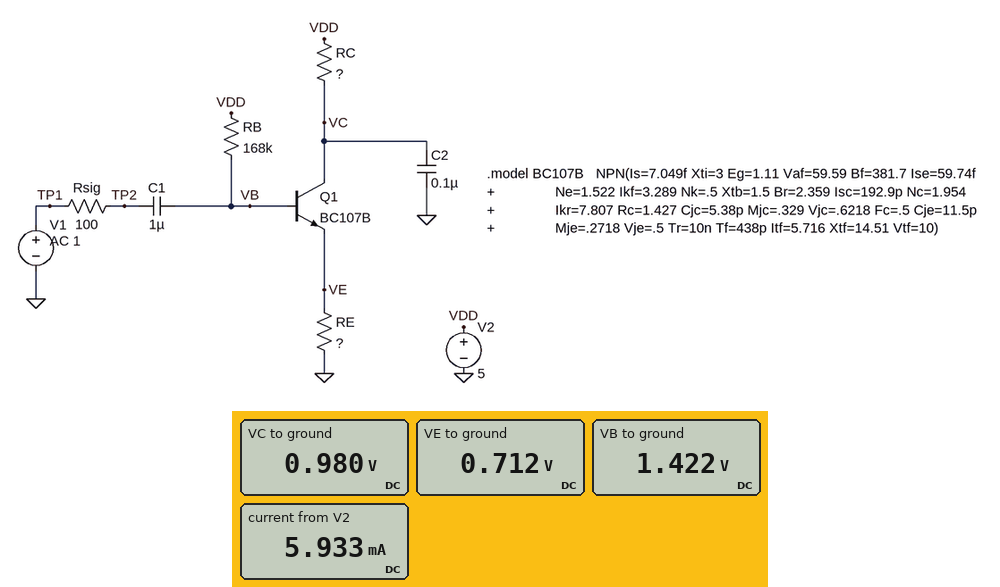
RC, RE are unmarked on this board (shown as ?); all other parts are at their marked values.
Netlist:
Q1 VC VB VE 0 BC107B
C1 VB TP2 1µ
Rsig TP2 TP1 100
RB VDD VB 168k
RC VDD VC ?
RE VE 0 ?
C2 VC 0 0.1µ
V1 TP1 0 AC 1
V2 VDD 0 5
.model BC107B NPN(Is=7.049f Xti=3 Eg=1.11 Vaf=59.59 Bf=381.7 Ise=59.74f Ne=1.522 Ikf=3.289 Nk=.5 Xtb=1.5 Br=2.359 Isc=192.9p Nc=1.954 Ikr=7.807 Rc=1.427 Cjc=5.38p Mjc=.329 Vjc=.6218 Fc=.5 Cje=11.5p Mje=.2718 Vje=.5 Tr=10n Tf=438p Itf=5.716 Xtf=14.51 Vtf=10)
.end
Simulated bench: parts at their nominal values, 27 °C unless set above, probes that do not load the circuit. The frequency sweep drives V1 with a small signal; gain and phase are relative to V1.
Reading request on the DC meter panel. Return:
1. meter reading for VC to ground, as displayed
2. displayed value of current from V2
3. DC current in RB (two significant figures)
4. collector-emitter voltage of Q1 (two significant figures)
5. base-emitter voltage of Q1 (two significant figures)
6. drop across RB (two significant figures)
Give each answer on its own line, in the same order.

0.980 V
5.933 mA
21 µA
270 mV
710 mV
3.6 V
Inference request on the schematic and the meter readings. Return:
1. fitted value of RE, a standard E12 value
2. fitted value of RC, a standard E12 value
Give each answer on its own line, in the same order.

120 Ω
680 Ω
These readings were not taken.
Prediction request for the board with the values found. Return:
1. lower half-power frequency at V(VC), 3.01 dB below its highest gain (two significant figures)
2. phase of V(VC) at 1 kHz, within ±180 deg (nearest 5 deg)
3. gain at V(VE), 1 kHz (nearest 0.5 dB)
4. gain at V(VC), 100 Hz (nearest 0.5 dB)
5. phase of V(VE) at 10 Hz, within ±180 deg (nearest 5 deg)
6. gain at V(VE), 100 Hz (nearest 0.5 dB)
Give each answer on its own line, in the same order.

37 Hz
160 deg
-0.5 dB
14.0 dB
75 deg
-1.0 dB
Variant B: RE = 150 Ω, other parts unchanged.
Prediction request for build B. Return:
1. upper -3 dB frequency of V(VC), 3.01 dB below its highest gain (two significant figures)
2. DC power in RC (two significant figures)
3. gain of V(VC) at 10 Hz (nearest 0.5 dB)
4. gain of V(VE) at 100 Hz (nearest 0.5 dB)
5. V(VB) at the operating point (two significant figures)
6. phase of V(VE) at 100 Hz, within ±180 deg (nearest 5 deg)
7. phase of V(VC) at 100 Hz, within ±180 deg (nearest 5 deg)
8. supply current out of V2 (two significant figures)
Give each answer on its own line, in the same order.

2.5 kHz
22 mW
3.0 dB
-0.5 dB
1.6 V
15 deg
-165 deg
5.7 mA
